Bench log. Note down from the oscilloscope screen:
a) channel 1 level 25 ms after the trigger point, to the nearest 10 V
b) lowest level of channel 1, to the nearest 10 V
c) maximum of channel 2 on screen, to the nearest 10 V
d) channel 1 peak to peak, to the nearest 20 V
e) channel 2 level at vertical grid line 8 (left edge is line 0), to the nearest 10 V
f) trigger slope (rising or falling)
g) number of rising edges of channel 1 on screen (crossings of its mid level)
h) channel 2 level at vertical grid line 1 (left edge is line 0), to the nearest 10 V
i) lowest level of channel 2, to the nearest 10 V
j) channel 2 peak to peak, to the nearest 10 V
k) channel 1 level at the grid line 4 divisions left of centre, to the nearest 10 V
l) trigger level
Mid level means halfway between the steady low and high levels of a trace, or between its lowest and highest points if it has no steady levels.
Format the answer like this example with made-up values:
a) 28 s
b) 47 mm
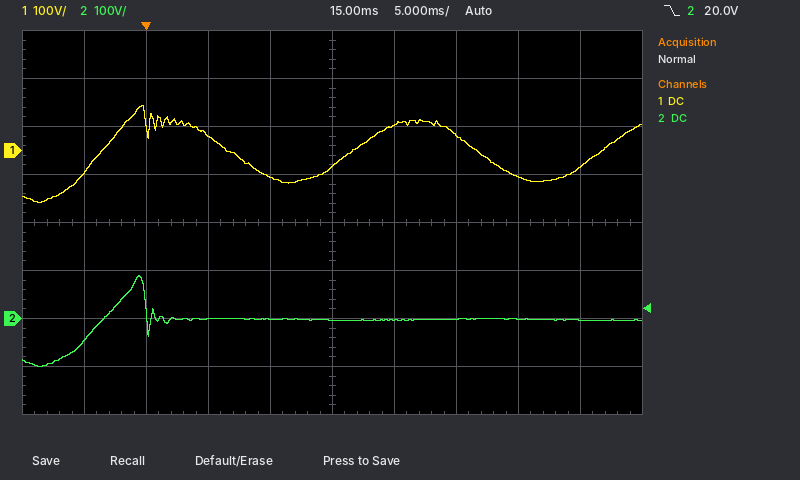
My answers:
a) 30 V
b) -110 V
c) 90 V
d) 200 V
e) 0 V
f) falling
g) 3
h) -50 V
i) -100 V
j) 190 V
k) -50 V
l) 20.0 V
